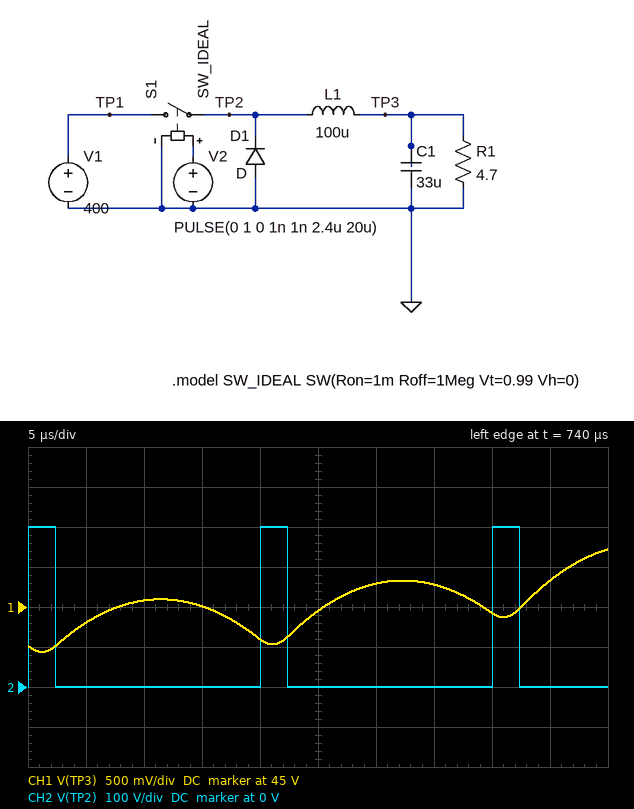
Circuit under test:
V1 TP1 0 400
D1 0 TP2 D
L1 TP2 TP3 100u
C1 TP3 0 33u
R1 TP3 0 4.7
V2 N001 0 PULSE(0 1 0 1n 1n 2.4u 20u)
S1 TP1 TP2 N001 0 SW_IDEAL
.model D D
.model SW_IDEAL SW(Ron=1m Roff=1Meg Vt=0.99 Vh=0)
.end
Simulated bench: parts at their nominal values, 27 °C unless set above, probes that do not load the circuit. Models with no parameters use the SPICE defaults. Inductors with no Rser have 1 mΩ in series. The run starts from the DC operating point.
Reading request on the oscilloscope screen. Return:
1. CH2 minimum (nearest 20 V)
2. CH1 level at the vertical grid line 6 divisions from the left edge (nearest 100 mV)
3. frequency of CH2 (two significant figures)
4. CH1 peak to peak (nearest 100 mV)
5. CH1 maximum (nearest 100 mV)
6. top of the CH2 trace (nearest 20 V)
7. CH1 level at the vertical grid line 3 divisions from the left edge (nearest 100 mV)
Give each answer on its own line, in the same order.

0 V
45.3 V
50 kHz
1.3 V
45.7 V
400 V
45.0 V
